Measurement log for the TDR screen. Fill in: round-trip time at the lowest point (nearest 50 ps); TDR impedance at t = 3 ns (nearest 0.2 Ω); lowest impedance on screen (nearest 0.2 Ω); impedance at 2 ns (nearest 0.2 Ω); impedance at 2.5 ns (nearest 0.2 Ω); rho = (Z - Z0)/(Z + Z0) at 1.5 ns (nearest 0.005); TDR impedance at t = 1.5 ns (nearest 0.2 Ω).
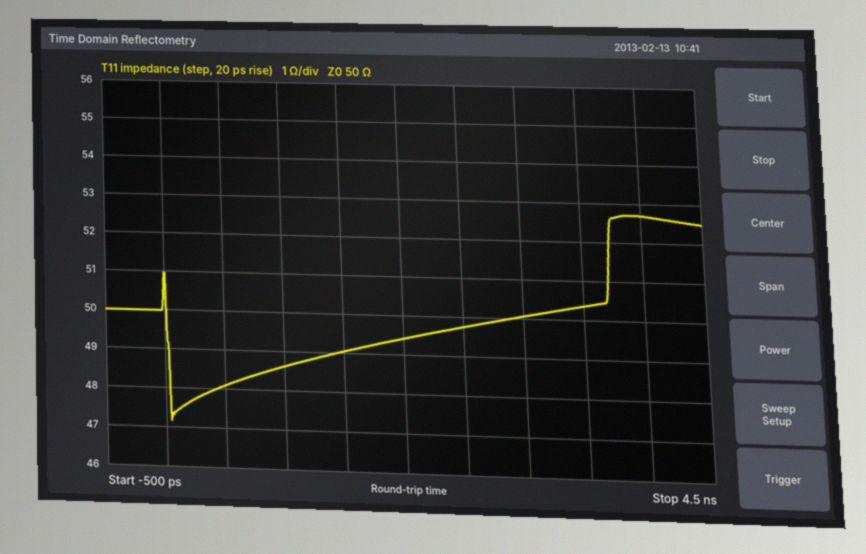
50 ps
50.0 Ω
47.2 Ω
49.4 Ω
49.8 Ω
-0.010
49.0 Ω
